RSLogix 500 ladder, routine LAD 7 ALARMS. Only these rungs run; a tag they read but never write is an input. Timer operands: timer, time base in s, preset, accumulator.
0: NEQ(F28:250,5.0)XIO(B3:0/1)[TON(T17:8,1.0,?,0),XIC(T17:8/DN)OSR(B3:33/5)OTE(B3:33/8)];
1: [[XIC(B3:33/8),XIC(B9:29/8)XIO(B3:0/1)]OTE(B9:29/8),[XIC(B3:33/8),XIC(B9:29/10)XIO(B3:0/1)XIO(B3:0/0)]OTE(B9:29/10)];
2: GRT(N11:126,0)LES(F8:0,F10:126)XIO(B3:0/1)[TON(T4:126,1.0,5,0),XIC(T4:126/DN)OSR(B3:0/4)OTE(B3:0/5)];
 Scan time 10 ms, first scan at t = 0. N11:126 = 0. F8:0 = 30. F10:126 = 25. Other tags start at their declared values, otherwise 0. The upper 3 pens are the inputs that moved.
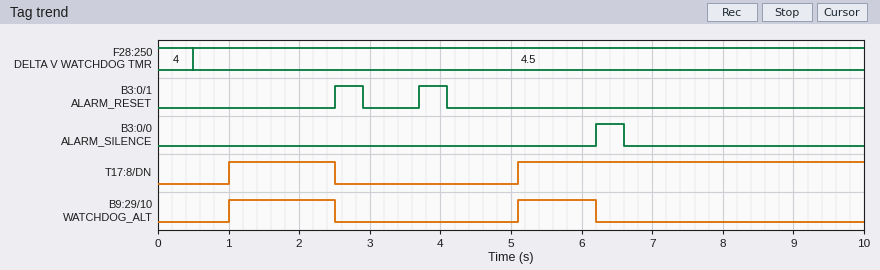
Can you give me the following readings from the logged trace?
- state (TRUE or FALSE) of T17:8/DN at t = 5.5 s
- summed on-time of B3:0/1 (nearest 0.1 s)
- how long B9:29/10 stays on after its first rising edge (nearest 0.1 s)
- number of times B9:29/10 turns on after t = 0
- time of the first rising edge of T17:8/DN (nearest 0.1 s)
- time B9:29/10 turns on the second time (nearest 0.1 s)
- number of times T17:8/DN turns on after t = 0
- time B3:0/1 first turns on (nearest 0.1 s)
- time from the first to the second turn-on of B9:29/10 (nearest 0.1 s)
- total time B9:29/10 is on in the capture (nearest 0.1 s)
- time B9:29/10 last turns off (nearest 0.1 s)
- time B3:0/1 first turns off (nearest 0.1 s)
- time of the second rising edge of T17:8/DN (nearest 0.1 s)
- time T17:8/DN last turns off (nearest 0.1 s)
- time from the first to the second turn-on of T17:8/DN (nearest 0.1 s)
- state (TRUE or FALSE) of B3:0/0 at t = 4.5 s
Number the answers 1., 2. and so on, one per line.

1. TRUE
2. 0.8 s
3. 1.5 s
4. 2
5. 1.0 s
6. 5.1 s
7. 2
8. 2.5 s
9. 4.1 s
10. 2.6 s
11. 6.2 s
12. 2.9 s
13. 5.1 s
14. 2.5 s
15. 4.1 s
16. FALSE
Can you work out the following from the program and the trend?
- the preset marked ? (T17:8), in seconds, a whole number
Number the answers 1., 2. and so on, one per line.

1. 1 s
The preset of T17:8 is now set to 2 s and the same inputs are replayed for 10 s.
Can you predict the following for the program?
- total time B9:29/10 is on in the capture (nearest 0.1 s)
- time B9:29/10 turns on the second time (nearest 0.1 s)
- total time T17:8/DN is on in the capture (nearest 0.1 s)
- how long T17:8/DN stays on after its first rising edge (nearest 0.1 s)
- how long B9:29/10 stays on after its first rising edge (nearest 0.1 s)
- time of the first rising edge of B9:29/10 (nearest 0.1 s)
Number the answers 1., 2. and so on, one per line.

1. 0.6 s
2. 6.1 s
3. 4.4 s
4. 0.5 s
5. 0.5 s
6. 2.0 s
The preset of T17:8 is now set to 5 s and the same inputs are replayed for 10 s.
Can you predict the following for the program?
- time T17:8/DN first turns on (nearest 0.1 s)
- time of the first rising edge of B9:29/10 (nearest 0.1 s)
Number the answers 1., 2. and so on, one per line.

1. 9.1 s
2. 9.1 s
